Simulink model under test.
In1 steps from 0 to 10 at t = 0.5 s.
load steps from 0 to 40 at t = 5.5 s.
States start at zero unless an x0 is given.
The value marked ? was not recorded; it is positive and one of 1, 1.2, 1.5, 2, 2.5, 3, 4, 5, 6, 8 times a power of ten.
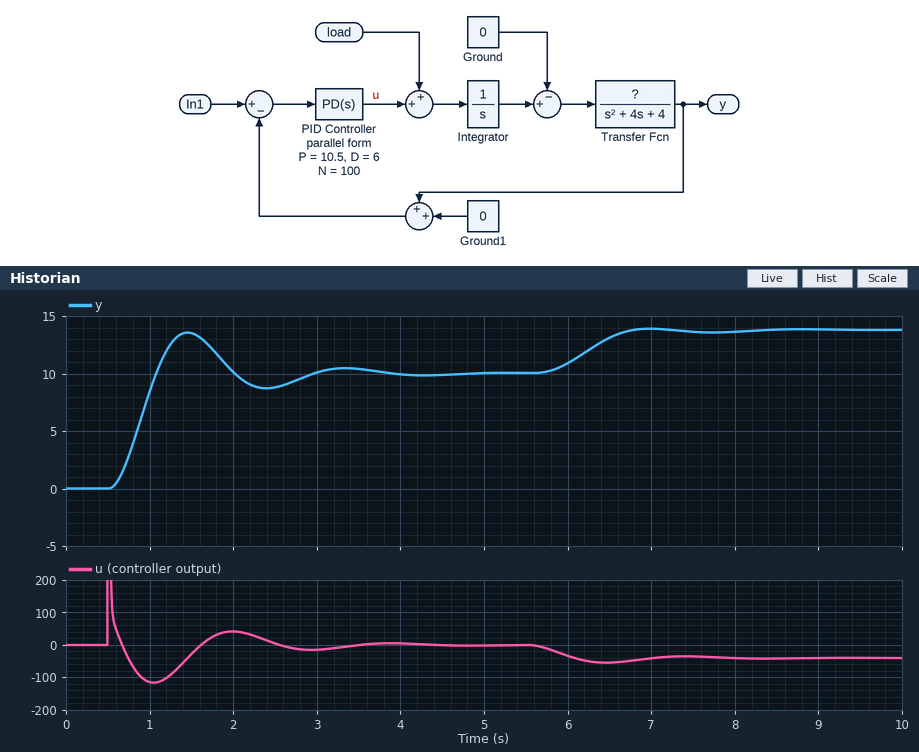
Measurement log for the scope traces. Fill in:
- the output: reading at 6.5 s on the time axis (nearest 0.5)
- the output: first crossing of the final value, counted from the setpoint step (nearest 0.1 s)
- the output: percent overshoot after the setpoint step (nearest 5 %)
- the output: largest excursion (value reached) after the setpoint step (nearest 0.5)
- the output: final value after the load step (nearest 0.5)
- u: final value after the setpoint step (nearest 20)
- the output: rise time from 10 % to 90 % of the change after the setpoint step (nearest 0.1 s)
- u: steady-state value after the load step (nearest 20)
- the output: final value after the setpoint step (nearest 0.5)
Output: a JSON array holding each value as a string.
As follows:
["13.0", "0.6 s", "35 %", "13.5", "14.0", "0", "0.4 s", "-40", "10.0"]
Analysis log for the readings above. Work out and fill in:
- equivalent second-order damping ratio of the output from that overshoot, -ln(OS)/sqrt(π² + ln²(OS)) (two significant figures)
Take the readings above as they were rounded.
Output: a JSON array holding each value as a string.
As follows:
["0.32"]
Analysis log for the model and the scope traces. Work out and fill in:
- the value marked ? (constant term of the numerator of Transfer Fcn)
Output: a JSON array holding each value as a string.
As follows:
["2"]
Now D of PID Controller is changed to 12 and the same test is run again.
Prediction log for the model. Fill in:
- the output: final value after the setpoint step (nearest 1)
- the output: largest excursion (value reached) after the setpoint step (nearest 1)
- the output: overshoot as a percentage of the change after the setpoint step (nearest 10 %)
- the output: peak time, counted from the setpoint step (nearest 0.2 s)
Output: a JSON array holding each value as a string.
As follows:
["10", "13", "30 %", "0.6 s"]
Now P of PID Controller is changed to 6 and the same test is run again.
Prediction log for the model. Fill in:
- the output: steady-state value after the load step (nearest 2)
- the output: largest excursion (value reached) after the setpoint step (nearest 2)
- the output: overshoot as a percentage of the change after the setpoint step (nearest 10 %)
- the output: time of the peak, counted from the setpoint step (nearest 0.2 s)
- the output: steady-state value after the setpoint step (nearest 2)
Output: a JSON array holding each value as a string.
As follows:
["16", "12", "20 %", "1.0 s", "10"]
